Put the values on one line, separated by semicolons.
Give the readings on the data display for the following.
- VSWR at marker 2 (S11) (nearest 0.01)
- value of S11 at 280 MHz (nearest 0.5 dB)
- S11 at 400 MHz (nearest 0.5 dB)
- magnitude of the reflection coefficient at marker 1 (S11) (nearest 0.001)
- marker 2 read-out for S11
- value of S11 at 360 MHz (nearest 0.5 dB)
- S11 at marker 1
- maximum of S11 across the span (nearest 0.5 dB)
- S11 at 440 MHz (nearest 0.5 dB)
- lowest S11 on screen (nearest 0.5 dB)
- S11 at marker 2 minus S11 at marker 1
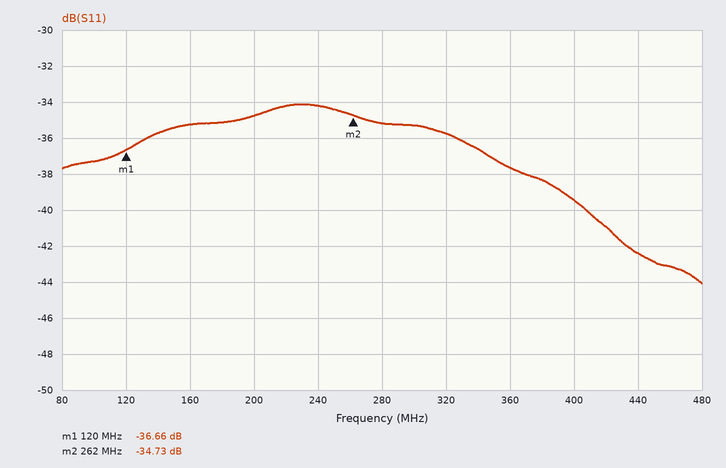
1.04; -35.0 dB; -39.5 dB; 0.015; -34.73 dB; -37.5 dB; -36.66 dB; -34.0 dB; -42.5 dB; -44.0 dB; 1.93 dB
